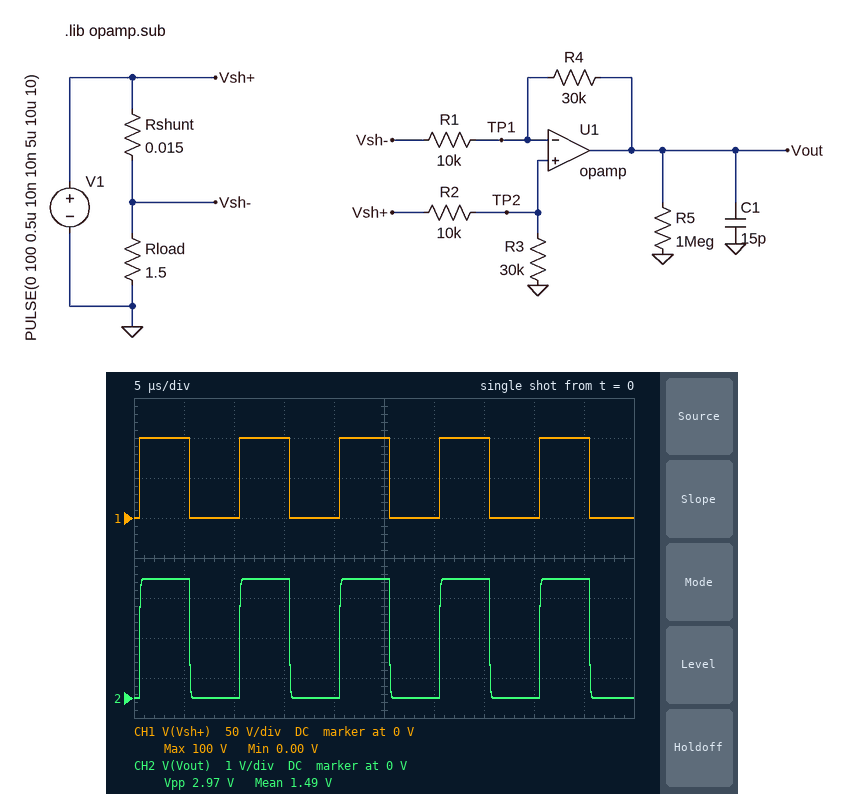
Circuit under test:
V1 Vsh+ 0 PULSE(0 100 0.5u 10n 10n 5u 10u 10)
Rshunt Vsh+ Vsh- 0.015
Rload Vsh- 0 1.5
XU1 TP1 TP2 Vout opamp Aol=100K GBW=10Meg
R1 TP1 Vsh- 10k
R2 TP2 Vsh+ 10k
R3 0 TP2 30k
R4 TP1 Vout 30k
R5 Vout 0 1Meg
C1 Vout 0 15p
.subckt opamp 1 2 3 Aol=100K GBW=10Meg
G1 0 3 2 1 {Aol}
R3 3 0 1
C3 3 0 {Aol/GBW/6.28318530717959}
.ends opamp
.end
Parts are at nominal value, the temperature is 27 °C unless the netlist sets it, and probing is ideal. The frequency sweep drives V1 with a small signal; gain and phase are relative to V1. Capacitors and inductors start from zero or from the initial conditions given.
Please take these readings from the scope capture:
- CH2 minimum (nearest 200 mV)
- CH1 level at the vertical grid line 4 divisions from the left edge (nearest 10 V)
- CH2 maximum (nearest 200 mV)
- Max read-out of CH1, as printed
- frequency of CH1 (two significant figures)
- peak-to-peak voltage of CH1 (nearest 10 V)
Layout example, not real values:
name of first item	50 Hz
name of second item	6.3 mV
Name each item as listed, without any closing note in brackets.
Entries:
CH2 minimum	0 V
CH1 level at the vertical grid line 4 divisions from the left edge	0 V
CH2 maximum	3.0 V
Max read-out of CH1, as printed	100 V
frequency of CH1	100 kHz
peak-to-peak voltage of CH1	100 V
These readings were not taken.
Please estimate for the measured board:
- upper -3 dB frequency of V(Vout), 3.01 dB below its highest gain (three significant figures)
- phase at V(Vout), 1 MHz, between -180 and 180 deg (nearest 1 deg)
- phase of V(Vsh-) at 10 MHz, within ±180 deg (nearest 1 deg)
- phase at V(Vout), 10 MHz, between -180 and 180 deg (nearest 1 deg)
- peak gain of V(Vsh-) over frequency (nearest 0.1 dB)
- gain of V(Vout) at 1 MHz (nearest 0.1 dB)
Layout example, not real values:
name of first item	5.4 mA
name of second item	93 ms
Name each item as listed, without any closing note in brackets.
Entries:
upper -3 dB frequency of V(Vout), 3.01 dB below its highest gain	2.50 MHz
phase at V(Vout), 1 MHz, between -180 and 180 deg	-22 deg
phase of V(Vsh-) at 10 MHz, within ±180 deg	0 deg
phase at V(Vout), 10 MHz, between -180 and 180 deg	-76 deg
peak gain of V(Vsh-) over frequency	-0.1 dB
gain of V(Vout) at 1 MHz	-31.2 dB
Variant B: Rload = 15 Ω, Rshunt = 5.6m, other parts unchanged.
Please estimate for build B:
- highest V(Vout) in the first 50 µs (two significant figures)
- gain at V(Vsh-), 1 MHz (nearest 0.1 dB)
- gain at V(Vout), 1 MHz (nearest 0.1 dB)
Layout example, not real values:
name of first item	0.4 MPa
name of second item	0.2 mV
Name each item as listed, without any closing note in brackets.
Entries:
highest V(Vout) in the first 50 µs	110 mV
gain at V(Vsh-), 1 MHz	0 dB
gain at V(Vout), 1 MHz	-59.7 dB
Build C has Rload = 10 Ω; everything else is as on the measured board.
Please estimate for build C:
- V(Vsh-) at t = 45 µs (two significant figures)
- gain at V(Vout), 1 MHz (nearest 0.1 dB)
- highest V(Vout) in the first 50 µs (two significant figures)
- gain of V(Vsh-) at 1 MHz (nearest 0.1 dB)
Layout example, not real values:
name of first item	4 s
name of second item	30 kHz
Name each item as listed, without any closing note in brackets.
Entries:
V(Vsh-) at t = 45 µs	100 V
gain at V(Vout), 1 MHz	-47.6 dB
highest V(Vout) in the first 50 µs	450 mV
gain of V(Vsh-) at 1 MHz	0 dB
